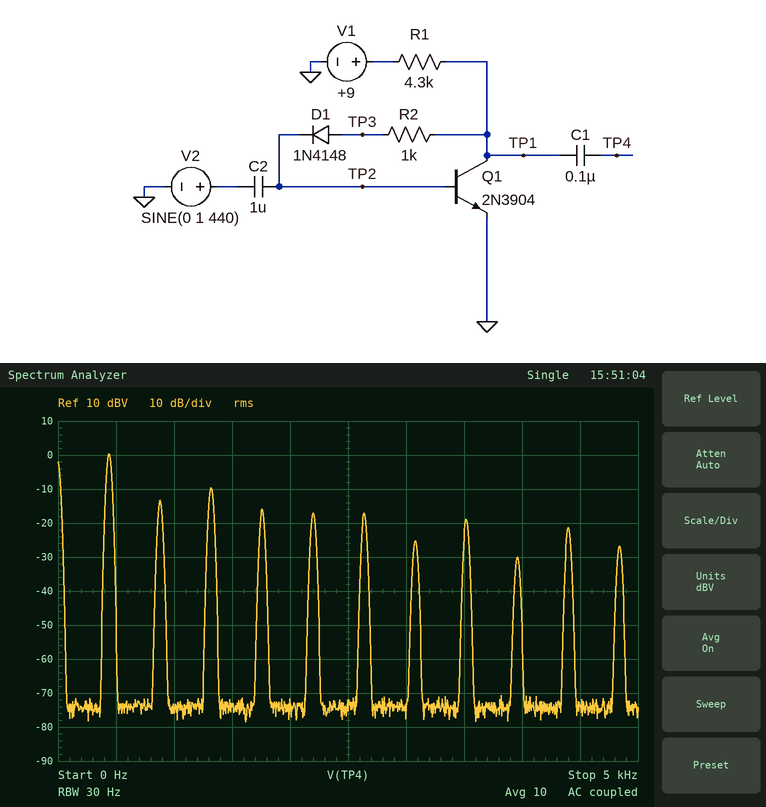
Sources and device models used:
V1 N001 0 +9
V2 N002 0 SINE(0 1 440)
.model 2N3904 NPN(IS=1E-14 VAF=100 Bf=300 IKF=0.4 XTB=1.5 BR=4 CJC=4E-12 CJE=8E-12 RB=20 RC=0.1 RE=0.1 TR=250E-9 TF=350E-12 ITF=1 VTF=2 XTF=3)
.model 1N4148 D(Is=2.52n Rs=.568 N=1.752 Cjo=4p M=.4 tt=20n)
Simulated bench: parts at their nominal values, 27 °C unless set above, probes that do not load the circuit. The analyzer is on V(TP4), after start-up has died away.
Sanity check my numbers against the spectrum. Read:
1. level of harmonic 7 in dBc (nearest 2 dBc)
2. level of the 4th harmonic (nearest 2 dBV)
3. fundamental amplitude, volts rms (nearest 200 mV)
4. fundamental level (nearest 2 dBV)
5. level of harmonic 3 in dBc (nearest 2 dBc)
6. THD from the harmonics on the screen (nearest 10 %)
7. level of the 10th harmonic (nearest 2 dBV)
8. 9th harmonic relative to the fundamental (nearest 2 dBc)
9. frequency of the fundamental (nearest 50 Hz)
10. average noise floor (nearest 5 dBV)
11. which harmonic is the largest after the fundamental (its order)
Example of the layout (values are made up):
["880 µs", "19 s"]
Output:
["-26 dBc", "-16 dBV", "1.0 V", "0 dBV", "-10 dBc", "50 %", "-22 dBV", "-30 dBc", "450 Hz", "-75 dBV", "3"]
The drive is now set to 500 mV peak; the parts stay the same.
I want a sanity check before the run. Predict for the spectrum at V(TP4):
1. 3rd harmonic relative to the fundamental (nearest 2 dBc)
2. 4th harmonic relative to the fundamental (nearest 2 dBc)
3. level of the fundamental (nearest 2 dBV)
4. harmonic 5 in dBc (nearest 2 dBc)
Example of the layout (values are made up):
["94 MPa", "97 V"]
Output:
["-14 dBc", "-22 dBc", "0 dBV", "-22 dBc"]
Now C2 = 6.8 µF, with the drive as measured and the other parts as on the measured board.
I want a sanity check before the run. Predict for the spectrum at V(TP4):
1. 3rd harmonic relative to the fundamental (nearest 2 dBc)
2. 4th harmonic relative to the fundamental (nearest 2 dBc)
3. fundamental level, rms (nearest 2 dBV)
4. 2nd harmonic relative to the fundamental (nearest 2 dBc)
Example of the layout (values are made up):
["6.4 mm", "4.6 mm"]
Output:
["-2 dBc", "-46 dBc", "-8 dBV", "4 dBc"]
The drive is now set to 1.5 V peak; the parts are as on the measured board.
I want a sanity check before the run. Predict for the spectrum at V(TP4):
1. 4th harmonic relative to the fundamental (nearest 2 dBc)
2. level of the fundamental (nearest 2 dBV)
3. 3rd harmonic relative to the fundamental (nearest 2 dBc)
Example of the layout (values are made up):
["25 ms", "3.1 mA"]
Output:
["-8 dBc", "-2 dBV", "-16 dBc"]
